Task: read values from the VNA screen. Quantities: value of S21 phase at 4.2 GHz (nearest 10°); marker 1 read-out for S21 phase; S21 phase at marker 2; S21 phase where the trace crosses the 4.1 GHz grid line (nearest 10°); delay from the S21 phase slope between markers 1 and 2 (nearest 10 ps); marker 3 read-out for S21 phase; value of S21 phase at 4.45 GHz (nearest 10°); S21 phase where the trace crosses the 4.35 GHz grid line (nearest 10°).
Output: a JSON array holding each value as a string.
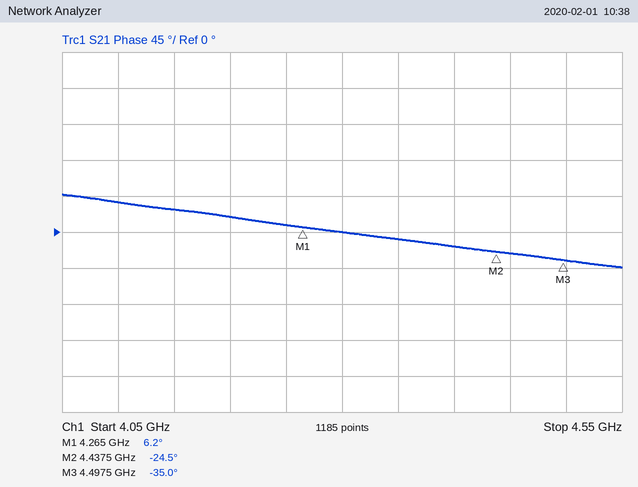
["20°", "6.2°", "-24.5°", "40°", "490 ps", "-35.0°", "-30°", "-10°"]
